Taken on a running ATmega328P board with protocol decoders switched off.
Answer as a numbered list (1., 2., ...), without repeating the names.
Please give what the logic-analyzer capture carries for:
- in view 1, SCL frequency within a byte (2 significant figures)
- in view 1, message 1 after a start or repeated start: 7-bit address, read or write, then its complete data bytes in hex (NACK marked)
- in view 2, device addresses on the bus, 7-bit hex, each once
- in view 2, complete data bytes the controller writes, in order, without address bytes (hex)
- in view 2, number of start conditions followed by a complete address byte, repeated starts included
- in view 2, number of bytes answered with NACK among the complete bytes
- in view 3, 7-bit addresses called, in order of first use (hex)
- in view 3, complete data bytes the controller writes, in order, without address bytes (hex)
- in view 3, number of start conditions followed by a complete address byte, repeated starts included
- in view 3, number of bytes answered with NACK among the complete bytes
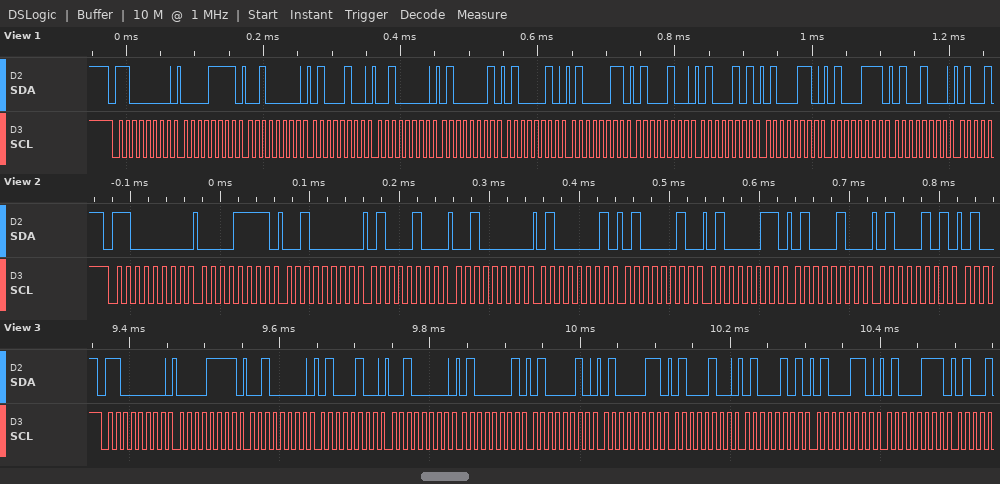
1. 100 kHz
2. 0x60 write: 0F 20 44 20 41 42 43 44 45 46 47 48
3. 0x60
4. 0F 20 44 20 41 42 43 44 45
5. 1
6. 0
7. 0x60
8. 0F 20 44 20 41 42 43 44 45 46 47
9. 1
10. 0
